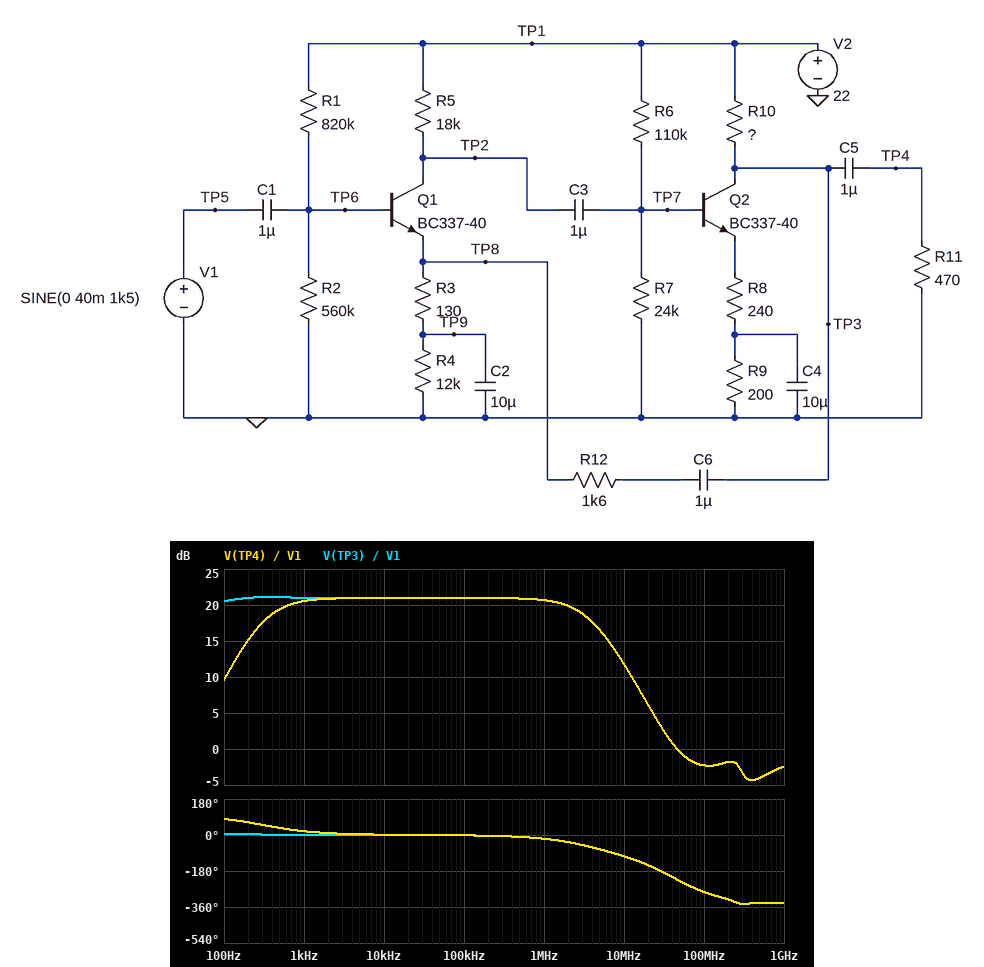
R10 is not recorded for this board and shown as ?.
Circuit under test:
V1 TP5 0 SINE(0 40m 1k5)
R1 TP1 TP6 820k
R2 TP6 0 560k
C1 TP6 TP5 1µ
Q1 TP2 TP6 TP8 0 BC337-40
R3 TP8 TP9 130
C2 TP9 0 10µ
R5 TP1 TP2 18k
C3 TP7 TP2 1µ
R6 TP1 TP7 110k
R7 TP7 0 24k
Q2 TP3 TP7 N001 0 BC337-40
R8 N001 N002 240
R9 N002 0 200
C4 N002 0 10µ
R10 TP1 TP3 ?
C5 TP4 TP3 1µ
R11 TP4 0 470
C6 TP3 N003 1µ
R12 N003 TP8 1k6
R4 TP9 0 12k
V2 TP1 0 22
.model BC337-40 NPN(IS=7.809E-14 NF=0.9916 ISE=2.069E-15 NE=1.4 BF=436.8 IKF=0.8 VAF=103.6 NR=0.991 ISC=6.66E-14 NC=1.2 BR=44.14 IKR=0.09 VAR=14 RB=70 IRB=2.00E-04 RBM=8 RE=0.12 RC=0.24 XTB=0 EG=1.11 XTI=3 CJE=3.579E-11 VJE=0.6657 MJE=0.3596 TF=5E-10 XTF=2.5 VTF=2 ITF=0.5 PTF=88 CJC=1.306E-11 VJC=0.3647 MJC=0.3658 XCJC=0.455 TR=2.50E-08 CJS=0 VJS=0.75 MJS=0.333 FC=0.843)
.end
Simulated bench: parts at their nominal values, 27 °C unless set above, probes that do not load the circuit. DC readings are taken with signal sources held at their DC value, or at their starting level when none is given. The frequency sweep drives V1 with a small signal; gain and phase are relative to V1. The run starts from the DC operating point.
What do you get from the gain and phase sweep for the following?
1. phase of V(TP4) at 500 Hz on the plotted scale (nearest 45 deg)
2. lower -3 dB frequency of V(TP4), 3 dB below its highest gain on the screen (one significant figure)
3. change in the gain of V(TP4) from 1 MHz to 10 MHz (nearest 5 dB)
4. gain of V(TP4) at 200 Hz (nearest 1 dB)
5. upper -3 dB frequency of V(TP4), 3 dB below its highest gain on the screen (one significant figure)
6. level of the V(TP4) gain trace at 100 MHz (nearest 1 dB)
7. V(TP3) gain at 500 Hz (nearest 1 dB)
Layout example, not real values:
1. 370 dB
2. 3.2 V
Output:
1. 45 deg
2. 300 Hz
3. -10 dB
4. 15 dB
5. 4 MHz
6. -2 dB
7. 21 dB
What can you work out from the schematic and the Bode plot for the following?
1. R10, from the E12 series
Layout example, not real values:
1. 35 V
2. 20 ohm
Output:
1. 2.7 kΩ
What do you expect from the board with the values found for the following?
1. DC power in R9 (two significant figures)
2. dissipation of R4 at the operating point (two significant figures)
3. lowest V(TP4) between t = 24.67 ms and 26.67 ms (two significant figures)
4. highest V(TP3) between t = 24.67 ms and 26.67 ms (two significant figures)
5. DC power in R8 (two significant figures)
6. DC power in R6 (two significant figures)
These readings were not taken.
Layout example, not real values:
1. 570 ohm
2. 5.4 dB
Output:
1. 9.1 mW
2. 5.0 mW
3. -430 mV
4. 4.3 V
5. 11 mW
6. 3.1 mW
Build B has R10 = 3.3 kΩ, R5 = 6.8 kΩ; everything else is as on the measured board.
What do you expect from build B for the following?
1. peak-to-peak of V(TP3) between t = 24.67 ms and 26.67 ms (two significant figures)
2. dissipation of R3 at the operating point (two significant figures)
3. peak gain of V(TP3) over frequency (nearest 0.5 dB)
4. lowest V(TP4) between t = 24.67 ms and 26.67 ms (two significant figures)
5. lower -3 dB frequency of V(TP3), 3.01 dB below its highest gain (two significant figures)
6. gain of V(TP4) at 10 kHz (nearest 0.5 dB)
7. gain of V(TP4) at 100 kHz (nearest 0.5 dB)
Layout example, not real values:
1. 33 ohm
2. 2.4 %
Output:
1. 650 mV
2. 55 µW
3. 8.5 dB
4. -290 mV
5. 64 Hz
6. 8.0 dB
7. 7.5 dB
